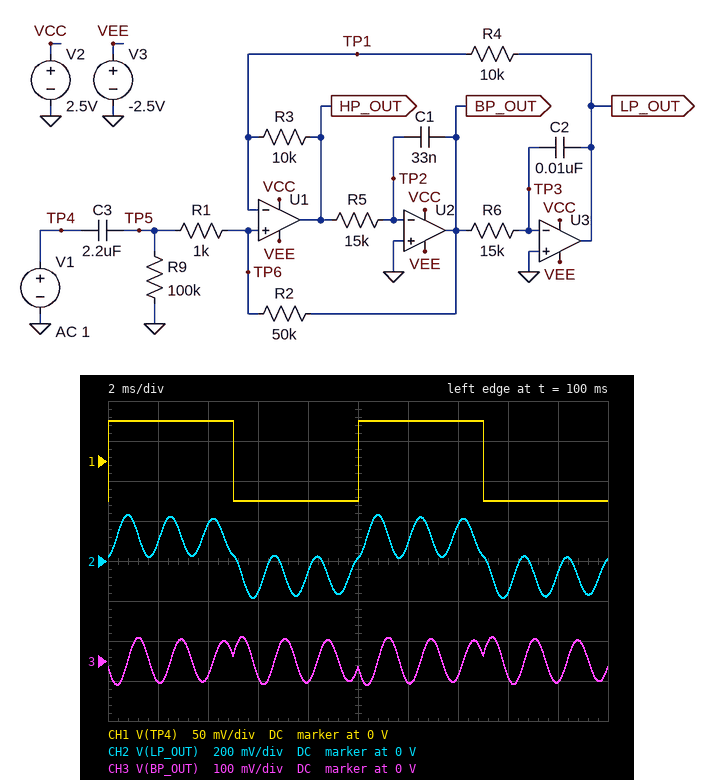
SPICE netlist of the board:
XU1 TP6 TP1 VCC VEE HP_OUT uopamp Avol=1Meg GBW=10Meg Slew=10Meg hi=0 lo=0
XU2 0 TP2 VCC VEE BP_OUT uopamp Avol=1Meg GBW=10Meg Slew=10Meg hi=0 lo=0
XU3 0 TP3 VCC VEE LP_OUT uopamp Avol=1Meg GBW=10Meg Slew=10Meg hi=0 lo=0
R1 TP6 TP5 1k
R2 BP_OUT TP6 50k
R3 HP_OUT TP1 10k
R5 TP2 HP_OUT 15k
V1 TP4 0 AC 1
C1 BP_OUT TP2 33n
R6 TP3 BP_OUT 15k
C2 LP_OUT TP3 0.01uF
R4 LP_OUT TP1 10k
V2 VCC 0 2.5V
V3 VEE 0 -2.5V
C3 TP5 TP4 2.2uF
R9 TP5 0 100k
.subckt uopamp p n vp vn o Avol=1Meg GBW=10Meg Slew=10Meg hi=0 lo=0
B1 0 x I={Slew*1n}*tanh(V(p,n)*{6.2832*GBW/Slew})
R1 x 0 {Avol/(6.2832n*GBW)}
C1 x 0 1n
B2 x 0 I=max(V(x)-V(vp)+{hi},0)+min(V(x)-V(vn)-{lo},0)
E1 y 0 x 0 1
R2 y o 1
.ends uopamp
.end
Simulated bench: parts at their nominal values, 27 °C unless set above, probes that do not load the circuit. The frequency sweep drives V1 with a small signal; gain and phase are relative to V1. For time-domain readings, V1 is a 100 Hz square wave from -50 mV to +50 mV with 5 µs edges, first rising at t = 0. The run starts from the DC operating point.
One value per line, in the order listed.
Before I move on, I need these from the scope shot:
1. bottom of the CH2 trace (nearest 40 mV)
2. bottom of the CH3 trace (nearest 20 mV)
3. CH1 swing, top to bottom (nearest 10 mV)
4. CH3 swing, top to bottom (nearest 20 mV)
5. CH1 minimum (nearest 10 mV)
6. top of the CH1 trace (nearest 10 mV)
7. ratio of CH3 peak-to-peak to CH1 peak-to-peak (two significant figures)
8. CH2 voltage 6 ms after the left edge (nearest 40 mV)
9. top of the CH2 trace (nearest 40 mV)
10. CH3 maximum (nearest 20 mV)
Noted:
-200 mV
-60 mV
100 mV
120 mV
-50 mV
50 mV
1.2
-160 mV
240 mV
60 mV
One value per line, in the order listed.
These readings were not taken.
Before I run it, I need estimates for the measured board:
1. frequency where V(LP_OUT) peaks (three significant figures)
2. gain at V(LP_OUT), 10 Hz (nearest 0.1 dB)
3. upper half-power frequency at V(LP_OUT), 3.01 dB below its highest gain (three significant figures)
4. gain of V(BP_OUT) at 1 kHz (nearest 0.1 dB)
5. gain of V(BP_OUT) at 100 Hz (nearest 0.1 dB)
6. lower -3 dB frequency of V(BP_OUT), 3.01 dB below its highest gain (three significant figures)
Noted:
585 Hz
5.6 dB
591 Hz
-0.4 dB
-14.4 dB
579 Hz
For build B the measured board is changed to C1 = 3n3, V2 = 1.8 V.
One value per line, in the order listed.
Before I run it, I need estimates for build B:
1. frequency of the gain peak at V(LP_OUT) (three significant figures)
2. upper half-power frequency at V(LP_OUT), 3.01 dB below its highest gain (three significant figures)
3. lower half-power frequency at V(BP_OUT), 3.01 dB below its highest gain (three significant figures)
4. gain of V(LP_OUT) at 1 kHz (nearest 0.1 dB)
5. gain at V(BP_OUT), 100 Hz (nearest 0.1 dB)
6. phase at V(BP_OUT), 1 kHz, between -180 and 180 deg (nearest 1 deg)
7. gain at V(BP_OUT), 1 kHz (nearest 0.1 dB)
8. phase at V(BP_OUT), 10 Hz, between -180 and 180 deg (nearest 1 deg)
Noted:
1.85 kHz
1.91 kHz
1.79 kHz
8.8 dB
-14.7 dB
-93 deg
8.3 dB
-78 deg
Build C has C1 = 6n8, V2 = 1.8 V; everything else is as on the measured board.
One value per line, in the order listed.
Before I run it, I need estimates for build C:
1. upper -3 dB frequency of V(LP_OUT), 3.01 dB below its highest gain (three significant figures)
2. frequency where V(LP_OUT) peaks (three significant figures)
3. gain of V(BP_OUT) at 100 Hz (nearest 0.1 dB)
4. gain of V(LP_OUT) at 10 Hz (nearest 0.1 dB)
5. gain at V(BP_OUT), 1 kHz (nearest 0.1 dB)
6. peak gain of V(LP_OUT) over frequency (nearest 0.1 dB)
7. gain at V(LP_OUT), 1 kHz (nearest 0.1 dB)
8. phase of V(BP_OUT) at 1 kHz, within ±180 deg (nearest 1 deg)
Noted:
1.32 kHz
1.29 kHz
-14.6 dB
5.6 dB
13.3 dB
32.4 dB
13.8 dB
-95 deg
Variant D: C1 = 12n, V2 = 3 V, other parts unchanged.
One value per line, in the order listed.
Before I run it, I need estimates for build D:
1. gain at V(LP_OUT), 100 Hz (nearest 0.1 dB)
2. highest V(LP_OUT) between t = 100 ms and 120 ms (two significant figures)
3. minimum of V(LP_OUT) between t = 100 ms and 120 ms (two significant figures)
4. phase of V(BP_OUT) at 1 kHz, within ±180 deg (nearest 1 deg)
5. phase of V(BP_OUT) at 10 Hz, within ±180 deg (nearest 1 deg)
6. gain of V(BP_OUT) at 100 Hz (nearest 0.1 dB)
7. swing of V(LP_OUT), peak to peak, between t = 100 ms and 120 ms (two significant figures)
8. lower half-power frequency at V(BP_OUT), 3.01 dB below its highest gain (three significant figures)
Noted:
5.9 dB
260 mV
-210 mV
120 deg
-78 deg
-14.6 dB
470 mV
953 Hz
